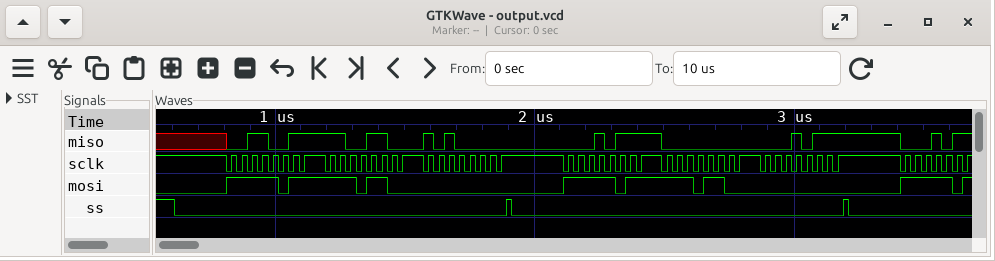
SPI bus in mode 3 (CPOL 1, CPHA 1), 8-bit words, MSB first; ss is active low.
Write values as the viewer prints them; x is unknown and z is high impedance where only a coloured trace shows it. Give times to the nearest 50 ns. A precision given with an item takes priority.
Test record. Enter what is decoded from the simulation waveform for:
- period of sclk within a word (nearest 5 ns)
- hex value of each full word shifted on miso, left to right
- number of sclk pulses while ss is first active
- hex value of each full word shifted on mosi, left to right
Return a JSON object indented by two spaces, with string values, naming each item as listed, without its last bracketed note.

{
  "period of sclk within a word": "40 ns",
  "hex value of each full word shifted on miso, left to right": "33, CC, A0, 17, 00, 17",
  "number of sclk pulses while ss is first active": "24",
  "hex value of each full word shifted on mosi, left to right": "FB, EC, 00, FB, EC, 00"
}
